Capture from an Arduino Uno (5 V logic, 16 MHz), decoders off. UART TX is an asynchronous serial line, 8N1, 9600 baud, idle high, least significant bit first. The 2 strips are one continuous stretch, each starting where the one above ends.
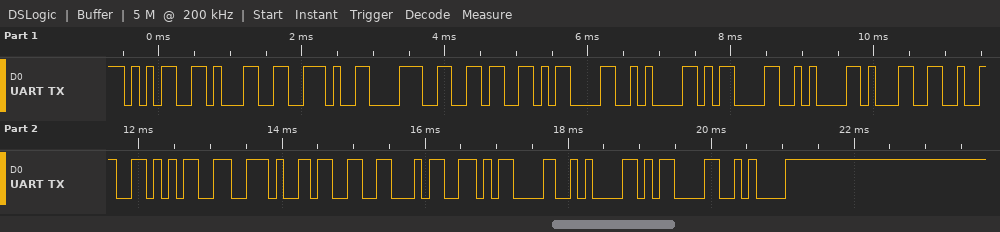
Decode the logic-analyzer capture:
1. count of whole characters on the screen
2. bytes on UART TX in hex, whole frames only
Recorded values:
19
35 31 2E 38 36 0D 0A 0D 0A 31 32 35 2E 33 34 0D 0A 0D 0A
